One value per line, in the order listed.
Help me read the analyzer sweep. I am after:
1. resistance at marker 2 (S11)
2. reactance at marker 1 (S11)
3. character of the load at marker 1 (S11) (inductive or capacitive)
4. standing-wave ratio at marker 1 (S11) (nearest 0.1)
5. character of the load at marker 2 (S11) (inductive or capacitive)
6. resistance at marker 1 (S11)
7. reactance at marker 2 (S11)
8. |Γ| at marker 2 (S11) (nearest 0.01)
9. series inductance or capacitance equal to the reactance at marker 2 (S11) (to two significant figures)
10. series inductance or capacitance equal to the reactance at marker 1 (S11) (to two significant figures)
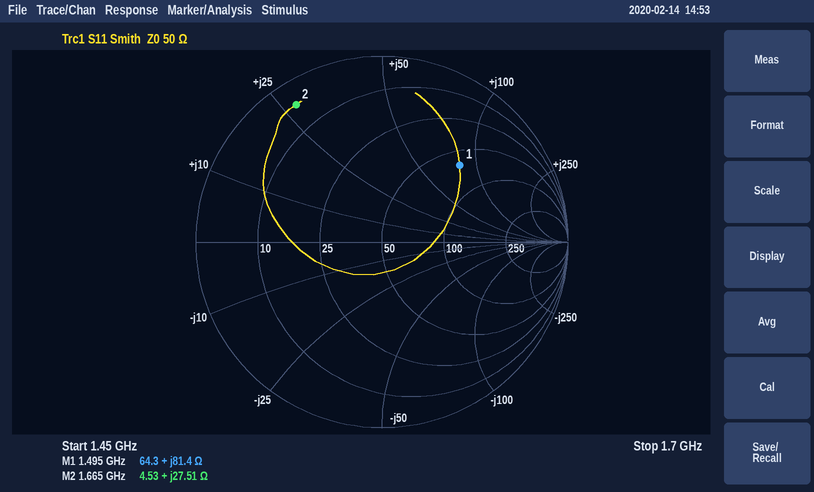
4.53 Ω
+81.4 Ω
inductive
3.9
inductive
64.3 Ω
+27.51 Ω
0.87
2.6 nH
8.7 nH
